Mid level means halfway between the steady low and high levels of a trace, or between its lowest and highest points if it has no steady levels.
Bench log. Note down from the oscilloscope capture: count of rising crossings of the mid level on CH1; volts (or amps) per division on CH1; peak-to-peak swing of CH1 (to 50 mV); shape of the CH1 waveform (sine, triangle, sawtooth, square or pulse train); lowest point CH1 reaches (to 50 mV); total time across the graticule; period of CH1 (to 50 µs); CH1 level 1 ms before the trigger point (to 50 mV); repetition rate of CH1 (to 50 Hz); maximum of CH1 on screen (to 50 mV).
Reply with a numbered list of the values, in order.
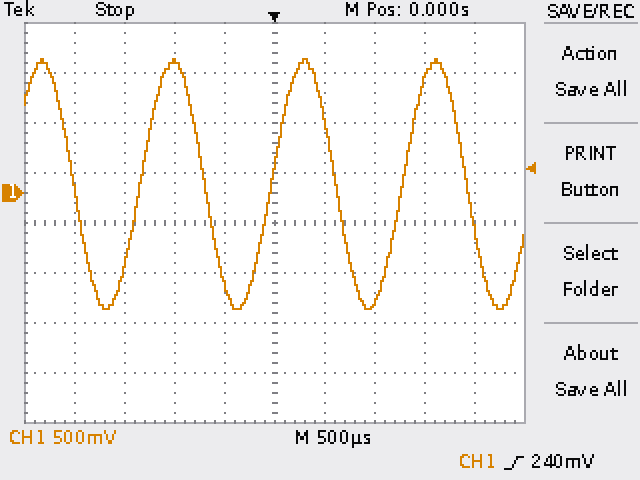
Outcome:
1. 3
2. 500 mV
3. 2.50 V
4. sine
5. -1.15 V
6. 5 ms
7. 1.30 ms
8. 1.30 V
9. 750 Hz
10. 1.35 V
